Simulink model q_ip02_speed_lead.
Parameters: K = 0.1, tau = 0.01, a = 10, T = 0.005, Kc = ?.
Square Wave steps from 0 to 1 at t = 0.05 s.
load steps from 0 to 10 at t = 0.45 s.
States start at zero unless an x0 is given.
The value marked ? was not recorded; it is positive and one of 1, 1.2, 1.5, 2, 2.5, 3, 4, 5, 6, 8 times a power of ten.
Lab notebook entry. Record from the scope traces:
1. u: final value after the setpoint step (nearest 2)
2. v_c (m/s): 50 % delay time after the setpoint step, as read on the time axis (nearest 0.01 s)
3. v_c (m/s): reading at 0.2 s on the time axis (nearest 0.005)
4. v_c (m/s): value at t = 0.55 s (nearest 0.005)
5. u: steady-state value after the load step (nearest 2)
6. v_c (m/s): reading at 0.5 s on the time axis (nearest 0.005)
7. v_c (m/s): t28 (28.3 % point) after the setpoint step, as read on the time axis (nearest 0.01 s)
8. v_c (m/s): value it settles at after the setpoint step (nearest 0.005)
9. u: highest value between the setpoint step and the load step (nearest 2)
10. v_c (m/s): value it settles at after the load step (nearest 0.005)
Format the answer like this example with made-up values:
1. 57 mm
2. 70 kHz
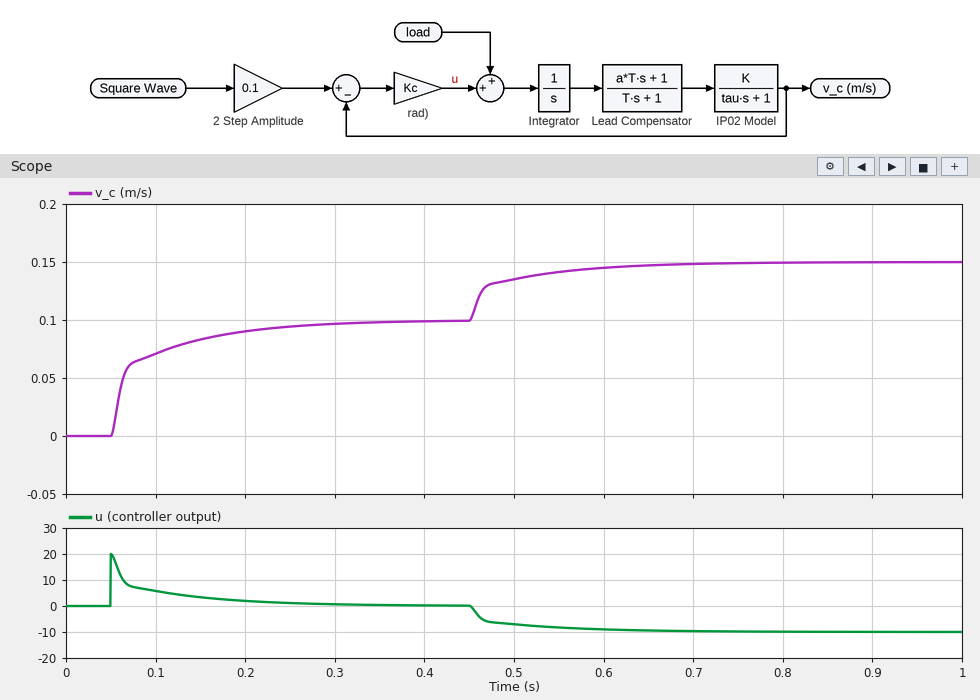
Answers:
1. 0
2. 0.06 s
3. 0.090
4. 0.140
5. -10
6. 0.135
7. 0.06 s
8. 0.100
9. 20
10. 0.150
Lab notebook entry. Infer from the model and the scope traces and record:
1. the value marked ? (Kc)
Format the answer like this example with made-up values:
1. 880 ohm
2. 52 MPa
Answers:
1. 200
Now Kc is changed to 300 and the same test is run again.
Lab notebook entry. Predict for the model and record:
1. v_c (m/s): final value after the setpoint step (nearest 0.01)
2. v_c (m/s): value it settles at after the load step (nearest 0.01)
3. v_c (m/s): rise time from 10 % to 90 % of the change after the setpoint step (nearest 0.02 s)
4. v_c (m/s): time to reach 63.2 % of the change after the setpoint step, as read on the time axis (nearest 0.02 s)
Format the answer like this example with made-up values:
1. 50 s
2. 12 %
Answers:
1. 0.10
2. 0.13
3. 0.10 s
4. 0.06 s
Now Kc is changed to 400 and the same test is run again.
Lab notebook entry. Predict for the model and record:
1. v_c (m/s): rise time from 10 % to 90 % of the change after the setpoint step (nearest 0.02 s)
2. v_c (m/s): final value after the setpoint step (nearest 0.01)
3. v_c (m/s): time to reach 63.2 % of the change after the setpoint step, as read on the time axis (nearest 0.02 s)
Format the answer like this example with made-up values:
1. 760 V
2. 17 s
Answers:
1. 0.08 s
2. 0.10
3. 0.06 s
